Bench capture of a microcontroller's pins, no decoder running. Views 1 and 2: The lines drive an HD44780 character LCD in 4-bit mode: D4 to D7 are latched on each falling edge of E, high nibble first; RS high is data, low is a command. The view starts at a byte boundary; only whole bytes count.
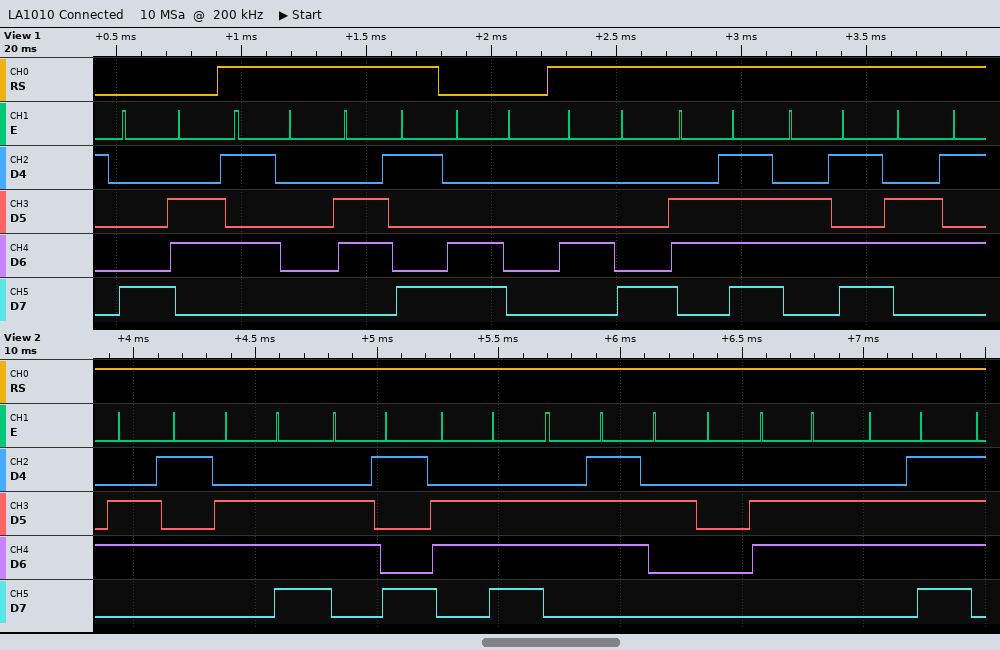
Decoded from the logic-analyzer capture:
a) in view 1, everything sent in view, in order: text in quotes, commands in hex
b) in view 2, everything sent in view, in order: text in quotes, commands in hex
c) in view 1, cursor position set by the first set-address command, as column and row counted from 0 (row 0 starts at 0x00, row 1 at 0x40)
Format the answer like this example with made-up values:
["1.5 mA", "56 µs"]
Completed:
["0x86 \"Pi\" 0xC0 \"Home\"", "\"ening fo\"", "column 6, row 0"]
